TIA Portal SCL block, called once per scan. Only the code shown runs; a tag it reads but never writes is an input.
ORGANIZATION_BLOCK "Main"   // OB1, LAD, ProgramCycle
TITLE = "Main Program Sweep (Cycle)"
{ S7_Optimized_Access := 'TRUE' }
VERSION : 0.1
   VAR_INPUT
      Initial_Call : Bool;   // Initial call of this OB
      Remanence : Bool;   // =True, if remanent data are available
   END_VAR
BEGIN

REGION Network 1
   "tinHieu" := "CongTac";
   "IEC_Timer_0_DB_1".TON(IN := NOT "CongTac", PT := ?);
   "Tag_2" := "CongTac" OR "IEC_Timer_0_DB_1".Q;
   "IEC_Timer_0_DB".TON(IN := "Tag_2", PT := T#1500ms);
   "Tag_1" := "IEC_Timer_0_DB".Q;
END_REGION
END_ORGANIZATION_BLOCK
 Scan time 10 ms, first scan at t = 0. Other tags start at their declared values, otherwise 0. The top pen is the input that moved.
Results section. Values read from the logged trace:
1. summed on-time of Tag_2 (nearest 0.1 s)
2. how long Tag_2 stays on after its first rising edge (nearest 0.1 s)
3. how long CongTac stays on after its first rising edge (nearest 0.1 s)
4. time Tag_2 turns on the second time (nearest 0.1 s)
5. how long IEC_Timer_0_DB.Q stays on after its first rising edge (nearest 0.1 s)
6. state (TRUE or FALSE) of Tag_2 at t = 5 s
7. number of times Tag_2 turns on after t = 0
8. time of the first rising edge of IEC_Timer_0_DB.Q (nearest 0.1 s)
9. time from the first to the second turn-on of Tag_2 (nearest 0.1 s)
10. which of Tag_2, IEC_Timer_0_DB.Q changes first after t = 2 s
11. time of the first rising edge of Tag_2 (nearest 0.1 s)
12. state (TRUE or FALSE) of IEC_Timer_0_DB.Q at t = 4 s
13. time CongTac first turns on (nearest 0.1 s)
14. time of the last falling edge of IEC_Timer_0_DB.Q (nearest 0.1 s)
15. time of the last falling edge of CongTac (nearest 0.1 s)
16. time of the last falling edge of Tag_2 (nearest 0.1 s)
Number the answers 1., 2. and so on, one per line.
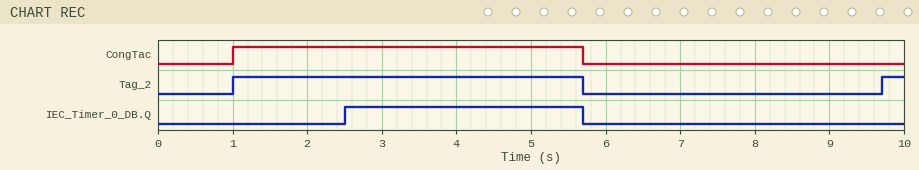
1. 5.0 s
2. 4.7 s
3. 4.7 s
4. 9.7 s
5. 3.2 s
6. TRUE
7. 2
8. 2.5 s
9. 8.7 s
10. IEC_Timer_0_DB.Q
11. 1.0 s
12. TRUE
13. 1.0 s
14. 5.7 s
15. 5.7 s
16. 5.7 s
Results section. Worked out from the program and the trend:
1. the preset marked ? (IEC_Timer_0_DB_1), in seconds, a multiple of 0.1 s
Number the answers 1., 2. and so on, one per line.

1. 4.0 s
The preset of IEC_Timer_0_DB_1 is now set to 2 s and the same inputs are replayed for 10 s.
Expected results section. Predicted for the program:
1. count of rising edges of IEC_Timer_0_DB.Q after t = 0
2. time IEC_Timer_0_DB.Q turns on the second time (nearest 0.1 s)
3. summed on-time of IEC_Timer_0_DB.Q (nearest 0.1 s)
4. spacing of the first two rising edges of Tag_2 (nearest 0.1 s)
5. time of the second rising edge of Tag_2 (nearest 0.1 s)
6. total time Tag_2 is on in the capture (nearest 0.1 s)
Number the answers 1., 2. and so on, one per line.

1. 2
2. 9.2 s
3. 4.0 s
4. 6.7 s
5. 7.7 s
6. 7.0 s
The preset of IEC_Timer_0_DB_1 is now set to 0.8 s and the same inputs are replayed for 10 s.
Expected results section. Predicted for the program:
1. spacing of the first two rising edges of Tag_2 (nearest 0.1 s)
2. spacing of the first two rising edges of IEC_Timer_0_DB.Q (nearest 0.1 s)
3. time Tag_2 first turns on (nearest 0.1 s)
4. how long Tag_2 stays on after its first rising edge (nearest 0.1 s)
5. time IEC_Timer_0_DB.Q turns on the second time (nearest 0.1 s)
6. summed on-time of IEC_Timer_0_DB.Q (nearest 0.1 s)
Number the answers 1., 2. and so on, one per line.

1. 5.7 s
2. 5.7 s
3. 0.8 s
4. 4.9 s
5. 8.0 s
6. 5.4 s
